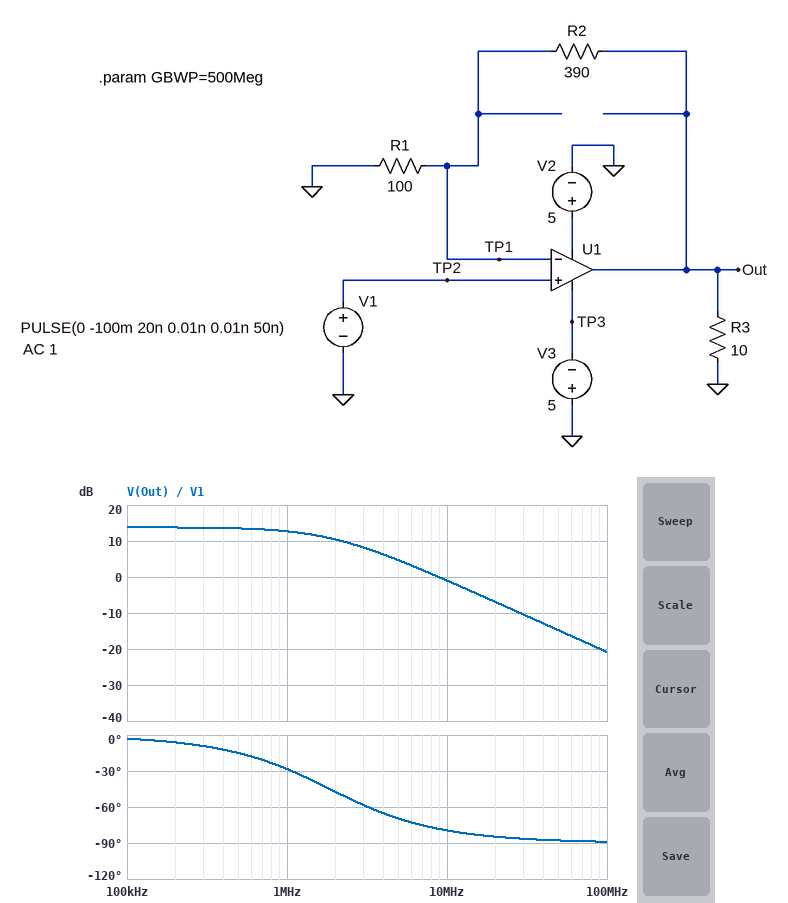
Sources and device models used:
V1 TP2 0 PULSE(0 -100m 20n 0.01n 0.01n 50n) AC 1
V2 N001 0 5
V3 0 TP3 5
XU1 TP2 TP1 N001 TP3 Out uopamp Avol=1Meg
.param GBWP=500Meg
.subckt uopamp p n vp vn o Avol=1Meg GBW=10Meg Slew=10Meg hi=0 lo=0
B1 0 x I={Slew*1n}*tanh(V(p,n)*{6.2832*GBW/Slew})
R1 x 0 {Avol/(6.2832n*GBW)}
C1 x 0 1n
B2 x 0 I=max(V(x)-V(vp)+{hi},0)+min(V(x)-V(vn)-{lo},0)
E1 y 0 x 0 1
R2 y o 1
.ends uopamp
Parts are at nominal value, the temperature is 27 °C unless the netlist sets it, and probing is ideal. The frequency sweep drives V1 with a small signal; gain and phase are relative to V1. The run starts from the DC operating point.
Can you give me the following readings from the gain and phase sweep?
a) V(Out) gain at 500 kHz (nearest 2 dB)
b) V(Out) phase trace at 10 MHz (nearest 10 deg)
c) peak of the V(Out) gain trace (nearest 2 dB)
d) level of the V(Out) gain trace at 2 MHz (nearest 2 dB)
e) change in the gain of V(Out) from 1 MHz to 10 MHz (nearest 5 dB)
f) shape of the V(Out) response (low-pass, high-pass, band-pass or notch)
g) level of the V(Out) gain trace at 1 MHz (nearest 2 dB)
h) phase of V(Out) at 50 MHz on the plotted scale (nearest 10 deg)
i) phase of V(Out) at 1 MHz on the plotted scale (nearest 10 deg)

14 dB
-80 deg
14 dB
10 dB
-15 dB
low-pass
12 dB
-90 deg
-30 deg
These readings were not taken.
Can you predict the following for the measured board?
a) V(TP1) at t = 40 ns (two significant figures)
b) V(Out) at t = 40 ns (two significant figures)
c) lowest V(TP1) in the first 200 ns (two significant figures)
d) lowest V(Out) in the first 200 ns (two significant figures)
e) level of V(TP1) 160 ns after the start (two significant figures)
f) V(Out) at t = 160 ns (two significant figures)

-19 mV
-93 mV
-42 mV
-200 mV
-15 mV
-72 mV
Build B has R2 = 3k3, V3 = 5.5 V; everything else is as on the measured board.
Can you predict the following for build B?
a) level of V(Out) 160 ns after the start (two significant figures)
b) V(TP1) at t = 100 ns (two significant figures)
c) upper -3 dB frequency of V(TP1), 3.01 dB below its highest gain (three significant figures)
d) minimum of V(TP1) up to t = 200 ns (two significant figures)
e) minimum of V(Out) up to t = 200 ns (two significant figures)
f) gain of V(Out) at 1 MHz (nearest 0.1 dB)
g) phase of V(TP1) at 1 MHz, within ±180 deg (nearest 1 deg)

-210 mV
-6.9 mV
267 kHz
-7.2 mV
-250 mV
18.9 dB
-75 deg
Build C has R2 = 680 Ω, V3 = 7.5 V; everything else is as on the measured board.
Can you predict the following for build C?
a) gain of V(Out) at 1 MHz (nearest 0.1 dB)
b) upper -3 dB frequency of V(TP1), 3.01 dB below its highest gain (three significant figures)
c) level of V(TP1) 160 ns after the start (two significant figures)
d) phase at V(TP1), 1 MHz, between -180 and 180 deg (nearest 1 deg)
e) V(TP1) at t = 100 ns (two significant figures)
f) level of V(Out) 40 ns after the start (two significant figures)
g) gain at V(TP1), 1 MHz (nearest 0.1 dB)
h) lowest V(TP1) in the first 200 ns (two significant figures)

15.4 dB
1.16 MHz
-15 mV
-41 deg
-23 mV
-96 mV
-2.4 dB
-28 mV
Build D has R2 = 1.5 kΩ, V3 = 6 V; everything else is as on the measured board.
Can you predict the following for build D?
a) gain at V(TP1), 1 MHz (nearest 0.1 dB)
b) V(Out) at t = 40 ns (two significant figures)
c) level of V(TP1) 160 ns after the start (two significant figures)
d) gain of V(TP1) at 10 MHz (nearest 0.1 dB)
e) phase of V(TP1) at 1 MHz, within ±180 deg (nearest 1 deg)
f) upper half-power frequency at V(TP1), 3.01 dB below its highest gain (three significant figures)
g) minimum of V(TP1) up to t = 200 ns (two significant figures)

-6.1 dB
-99 mV
-11 mV
-24.9 dB
-60 deg
568 kHz
-15 mV
